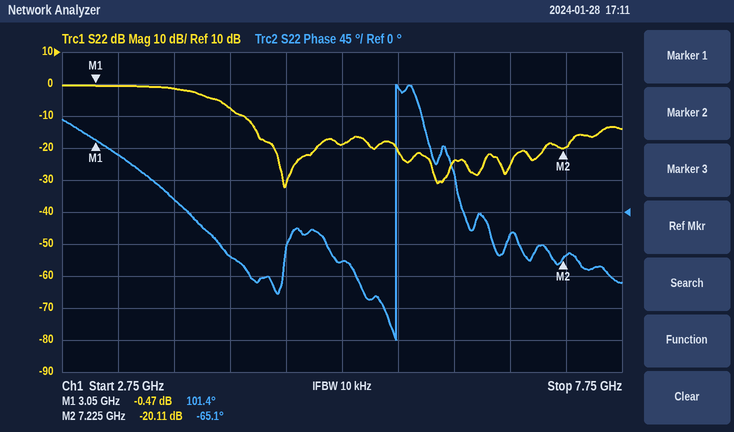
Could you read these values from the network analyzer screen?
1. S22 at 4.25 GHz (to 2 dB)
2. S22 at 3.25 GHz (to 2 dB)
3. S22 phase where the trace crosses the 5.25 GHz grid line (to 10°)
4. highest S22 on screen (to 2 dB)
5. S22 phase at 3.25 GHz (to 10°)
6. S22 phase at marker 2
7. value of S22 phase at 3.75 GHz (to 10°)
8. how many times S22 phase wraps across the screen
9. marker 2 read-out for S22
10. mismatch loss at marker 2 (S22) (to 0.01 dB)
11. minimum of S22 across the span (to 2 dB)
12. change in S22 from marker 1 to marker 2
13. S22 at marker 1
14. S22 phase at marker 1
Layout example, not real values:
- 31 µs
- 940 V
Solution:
- -8 dB
- 0 dB
- -70°
- 0 dB
- 80°
- -65.1°
- 20°
- 1
- -20.11 dB
- 0.04 dB
- -32 dB
- -19.64 dB
- -0.47 dB
- 101.4°
